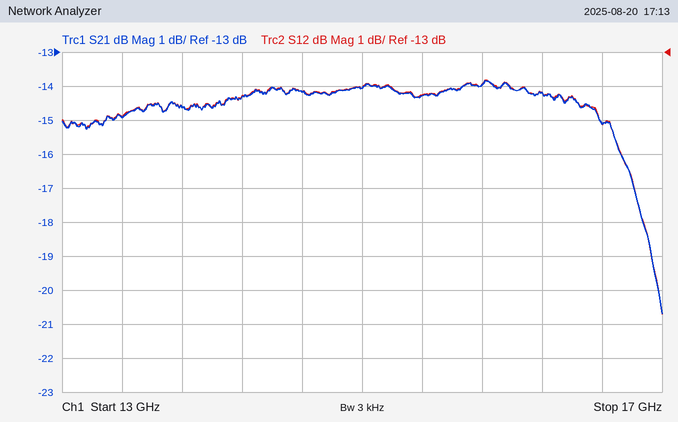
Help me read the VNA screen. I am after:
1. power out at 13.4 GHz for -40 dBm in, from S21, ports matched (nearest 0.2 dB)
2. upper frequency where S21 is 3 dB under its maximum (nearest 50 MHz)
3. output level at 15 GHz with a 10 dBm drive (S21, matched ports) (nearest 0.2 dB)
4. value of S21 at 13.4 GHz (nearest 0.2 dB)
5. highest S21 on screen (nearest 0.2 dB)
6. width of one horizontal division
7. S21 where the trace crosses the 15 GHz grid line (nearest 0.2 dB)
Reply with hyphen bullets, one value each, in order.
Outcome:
- -55.0 dBm
- 16.80 GHz
- -4.0 dBm
- -15.0 dB
- -13.8 dB
- 400 MHz
- -14.0 dB
